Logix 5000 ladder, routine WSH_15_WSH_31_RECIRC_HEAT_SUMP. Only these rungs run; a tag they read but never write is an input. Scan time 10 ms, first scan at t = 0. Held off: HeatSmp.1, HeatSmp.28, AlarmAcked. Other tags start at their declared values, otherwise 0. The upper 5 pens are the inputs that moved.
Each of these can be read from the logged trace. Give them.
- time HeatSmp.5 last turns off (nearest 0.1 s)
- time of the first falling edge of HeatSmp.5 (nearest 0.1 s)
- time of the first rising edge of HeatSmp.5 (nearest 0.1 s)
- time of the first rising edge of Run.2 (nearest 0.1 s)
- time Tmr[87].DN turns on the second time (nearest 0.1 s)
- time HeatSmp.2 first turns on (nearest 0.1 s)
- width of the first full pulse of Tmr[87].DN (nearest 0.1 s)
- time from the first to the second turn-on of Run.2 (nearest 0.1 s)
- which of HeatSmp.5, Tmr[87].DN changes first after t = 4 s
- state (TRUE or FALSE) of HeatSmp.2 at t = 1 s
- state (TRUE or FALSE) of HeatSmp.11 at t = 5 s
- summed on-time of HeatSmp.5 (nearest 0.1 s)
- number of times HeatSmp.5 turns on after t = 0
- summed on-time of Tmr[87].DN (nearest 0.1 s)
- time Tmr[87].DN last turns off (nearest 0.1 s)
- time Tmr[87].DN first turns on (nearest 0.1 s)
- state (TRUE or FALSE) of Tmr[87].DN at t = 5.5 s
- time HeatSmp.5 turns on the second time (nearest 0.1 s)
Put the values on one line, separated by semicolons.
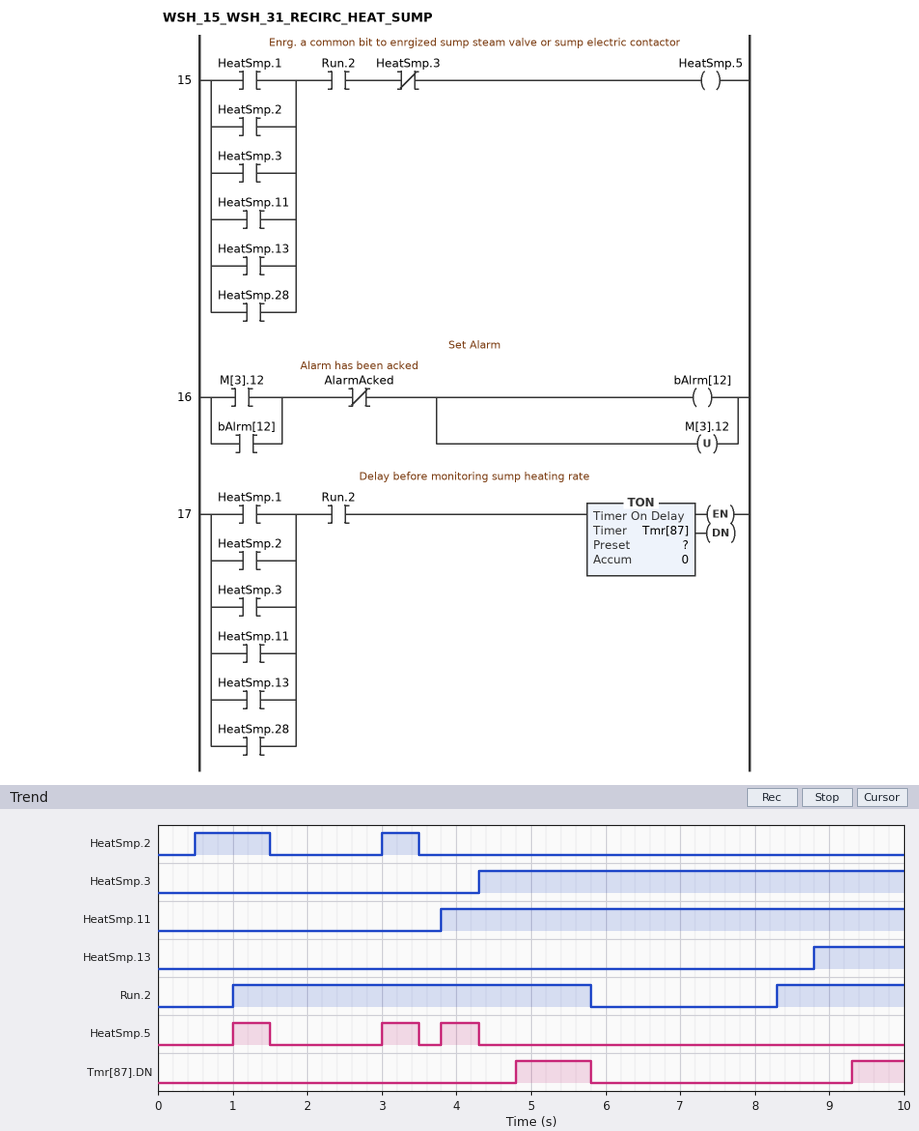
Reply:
4.3 s; 1.5 s; 1.0 s; 1.0 s; 9.3 s; 0.5 s; 1.0 s; 7.3 s; HeatSmp.5; TRUE; TRUE; 1.5 s; 3; 1.7 s; 5.8 s; 4.8 s; TRUE; 3.0 s
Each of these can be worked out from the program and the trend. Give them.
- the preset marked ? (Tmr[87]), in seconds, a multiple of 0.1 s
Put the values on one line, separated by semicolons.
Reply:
1.0 s
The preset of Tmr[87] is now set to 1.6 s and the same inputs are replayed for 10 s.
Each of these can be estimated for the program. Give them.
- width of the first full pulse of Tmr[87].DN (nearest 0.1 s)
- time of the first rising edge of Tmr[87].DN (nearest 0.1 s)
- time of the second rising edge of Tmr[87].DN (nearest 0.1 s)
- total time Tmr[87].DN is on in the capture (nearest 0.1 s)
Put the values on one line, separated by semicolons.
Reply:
0.4 s; 5.4 s; 9.9 s; 0.5 s
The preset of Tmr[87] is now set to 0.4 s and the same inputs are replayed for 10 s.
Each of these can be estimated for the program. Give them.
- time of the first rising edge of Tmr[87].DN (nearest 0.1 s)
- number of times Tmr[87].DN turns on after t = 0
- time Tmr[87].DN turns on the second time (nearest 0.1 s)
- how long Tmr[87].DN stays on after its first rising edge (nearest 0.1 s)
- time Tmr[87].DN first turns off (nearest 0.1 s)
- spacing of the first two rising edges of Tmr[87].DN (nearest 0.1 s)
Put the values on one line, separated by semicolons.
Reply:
1.4 s; 4; 3.4 s; 0.1 s; 1.5 s; 2.0 s
